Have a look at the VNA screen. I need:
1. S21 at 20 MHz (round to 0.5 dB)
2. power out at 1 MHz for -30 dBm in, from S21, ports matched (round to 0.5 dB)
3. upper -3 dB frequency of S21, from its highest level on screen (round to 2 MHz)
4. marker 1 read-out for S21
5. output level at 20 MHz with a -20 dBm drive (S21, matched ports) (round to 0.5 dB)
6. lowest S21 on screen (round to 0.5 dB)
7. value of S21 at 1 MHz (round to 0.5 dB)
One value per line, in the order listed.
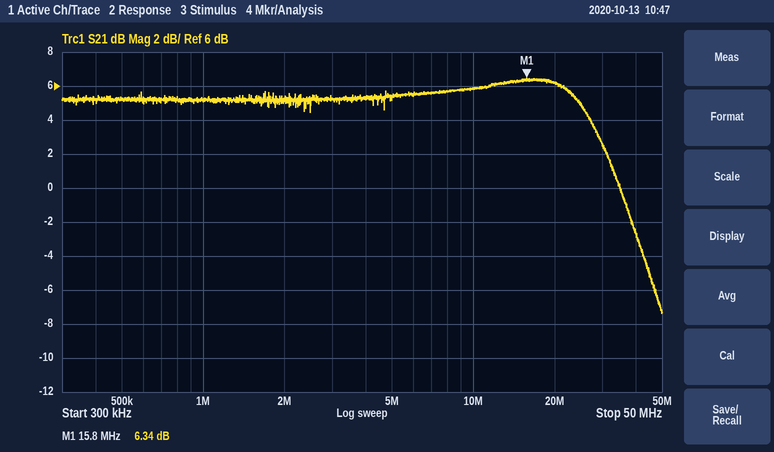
6.0 dB
-25.0 dBm
28 MHz
6.34 dB
-14.0 dBm
-7.5 dB
5.0 dB
